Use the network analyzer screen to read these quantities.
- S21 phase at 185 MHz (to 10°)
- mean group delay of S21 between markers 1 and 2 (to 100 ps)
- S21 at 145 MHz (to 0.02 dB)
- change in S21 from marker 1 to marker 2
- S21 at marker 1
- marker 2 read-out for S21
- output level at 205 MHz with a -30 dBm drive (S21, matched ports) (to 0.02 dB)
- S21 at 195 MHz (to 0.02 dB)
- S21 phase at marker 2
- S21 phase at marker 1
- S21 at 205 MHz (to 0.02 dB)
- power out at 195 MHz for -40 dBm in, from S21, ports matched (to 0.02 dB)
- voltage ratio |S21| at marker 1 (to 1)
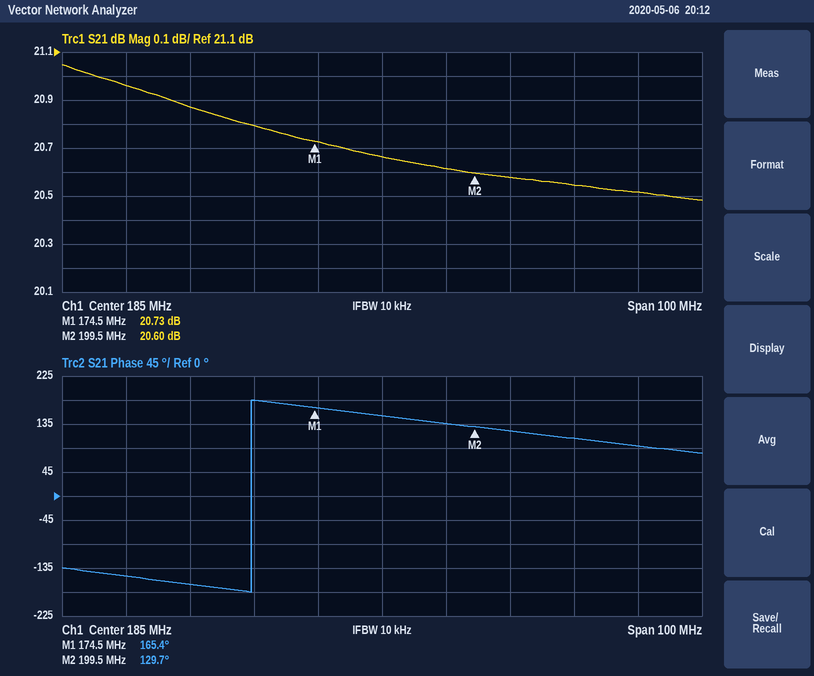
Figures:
150°
4.0 ns
20.96 dB
-0.13 dB
20.73 dB
20.60 dB
-9.42 dBm
20.62 dB
129.7°
165.4°
20.58 dB
-19.38 dBm
11
